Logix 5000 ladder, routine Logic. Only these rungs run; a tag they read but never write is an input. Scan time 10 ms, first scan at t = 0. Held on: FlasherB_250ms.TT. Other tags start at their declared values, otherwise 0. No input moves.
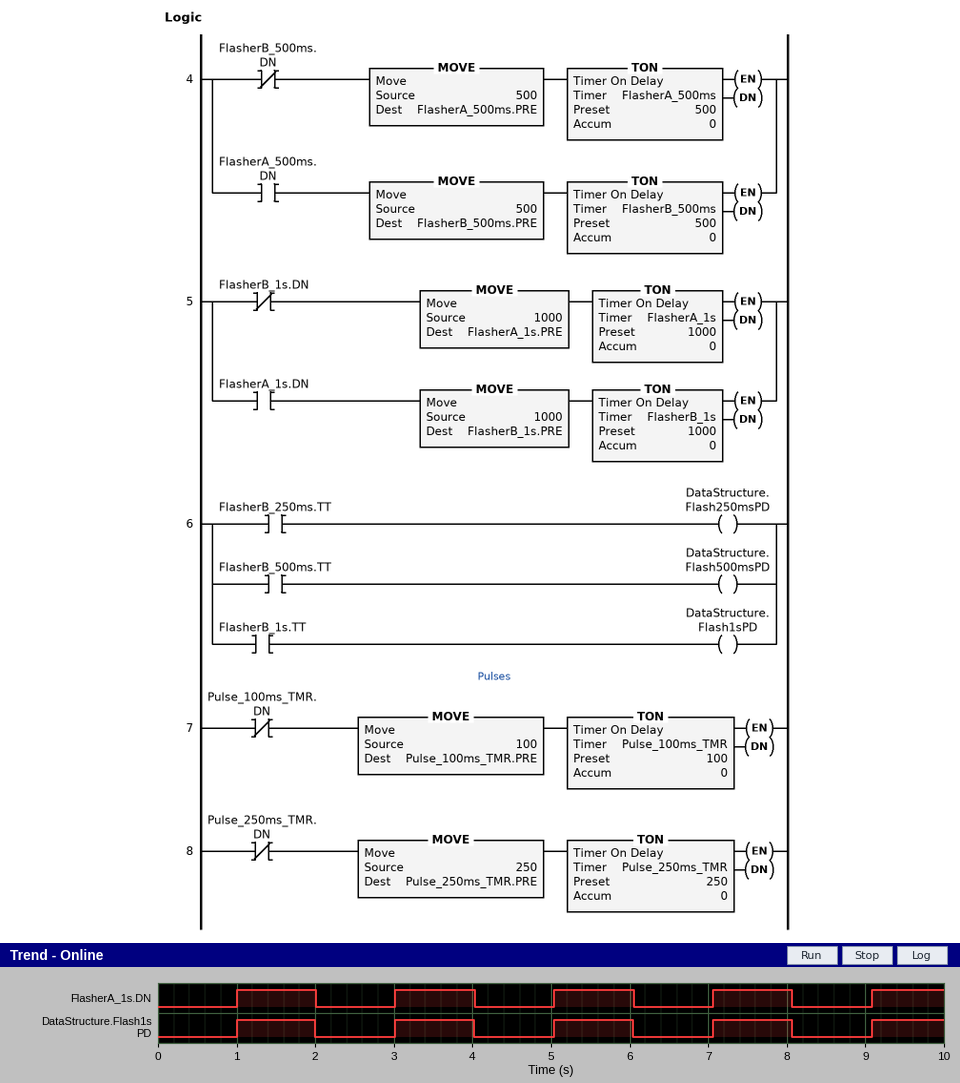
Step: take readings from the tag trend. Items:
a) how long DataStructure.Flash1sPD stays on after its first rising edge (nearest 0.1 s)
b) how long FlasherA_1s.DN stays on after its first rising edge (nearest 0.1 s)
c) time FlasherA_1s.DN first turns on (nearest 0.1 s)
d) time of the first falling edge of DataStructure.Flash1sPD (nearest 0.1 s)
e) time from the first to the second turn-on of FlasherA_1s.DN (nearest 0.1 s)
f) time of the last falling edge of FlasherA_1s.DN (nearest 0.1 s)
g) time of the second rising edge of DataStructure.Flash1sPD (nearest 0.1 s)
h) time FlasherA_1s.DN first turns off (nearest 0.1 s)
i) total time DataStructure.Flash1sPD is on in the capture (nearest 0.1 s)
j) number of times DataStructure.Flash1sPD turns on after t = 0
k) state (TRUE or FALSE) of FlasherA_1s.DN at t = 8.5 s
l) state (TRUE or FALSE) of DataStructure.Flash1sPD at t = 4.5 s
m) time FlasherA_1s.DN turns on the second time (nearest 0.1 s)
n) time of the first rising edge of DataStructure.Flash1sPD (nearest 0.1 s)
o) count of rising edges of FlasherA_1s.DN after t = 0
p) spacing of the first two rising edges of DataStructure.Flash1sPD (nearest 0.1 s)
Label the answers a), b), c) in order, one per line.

a) 1.0 s
b) 1.0 s
c) 1.0 s
d) 2.0 s
e) 2.0 s
f) 8.1 s
g) 3.0 s
h) 2.0 s
i) 4.9 s
j) 5
k) FALSE
l) FALSE
m) 3.0 s
n) 1.0 s
o) 5
p) 2.0 s
